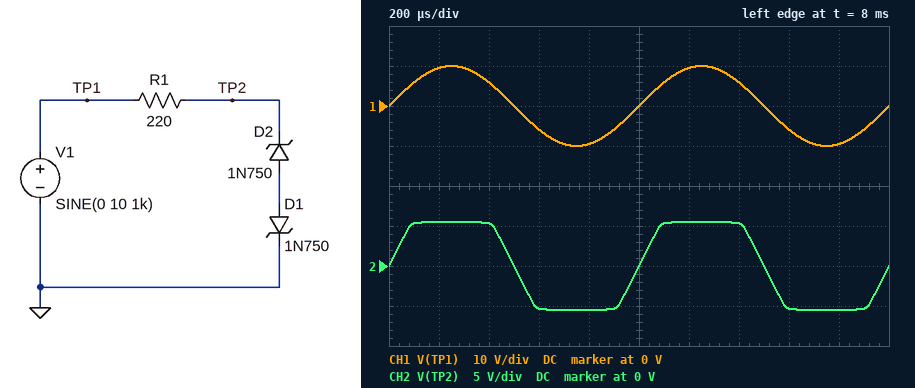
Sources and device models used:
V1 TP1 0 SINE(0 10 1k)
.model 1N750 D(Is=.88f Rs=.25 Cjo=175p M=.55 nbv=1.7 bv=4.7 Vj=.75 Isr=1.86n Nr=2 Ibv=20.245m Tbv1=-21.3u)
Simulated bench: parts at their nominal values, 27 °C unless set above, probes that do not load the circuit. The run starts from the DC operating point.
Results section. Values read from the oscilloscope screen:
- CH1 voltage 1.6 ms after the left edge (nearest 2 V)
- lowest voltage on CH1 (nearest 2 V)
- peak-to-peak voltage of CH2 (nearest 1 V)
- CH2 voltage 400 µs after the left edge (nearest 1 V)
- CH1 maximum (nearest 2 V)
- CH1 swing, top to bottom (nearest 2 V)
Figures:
-6 V
-10 V
11 V
5 V
10 V
20 V
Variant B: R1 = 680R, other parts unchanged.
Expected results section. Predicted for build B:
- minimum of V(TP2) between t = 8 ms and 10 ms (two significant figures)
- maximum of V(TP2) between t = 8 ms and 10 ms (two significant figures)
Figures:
-5.4 V
5.4 V
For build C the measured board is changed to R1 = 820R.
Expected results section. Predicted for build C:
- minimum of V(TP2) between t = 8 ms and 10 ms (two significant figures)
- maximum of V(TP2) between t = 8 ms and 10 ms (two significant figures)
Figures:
-5.4 V
5.4 V
